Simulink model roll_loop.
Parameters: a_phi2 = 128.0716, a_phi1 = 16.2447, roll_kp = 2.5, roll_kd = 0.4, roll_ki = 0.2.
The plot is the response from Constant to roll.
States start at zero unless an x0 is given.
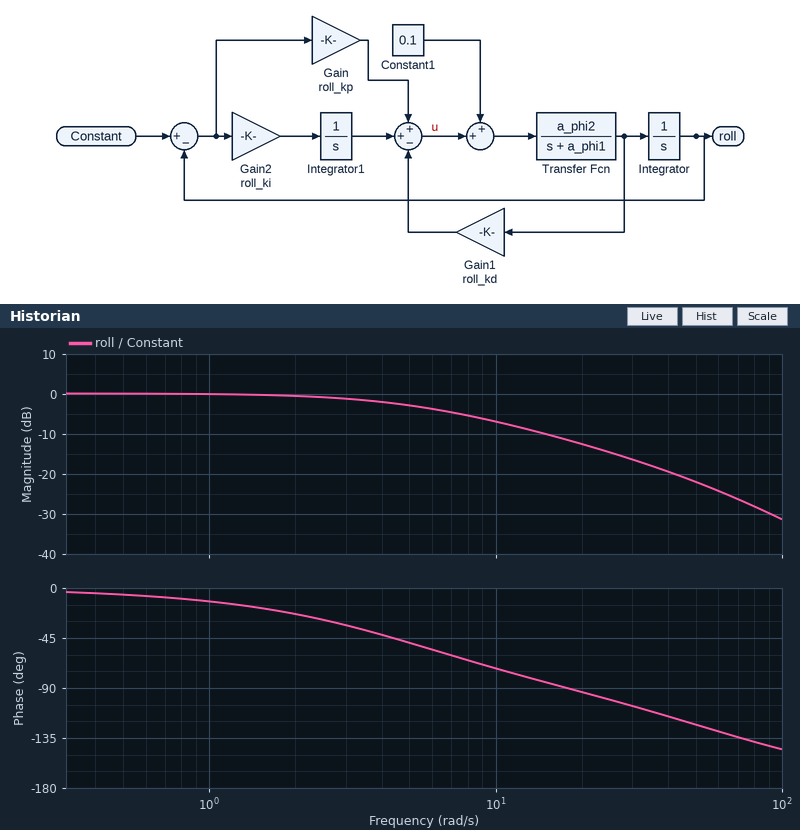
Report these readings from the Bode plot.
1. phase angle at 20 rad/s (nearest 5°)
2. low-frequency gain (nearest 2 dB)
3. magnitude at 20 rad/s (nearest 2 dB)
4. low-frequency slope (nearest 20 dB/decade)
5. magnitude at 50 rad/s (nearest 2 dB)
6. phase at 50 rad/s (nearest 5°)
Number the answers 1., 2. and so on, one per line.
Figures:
1. -95°
2. 0 dB
3. -12 dB
4. 0 dB/decade
5. -22 dB
6. -125°
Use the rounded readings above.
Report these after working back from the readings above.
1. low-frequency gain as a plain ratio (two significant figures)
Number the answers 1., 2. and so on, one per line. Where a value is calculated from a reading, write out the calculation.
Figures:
1. 10^(0 / 20) = 1.0
